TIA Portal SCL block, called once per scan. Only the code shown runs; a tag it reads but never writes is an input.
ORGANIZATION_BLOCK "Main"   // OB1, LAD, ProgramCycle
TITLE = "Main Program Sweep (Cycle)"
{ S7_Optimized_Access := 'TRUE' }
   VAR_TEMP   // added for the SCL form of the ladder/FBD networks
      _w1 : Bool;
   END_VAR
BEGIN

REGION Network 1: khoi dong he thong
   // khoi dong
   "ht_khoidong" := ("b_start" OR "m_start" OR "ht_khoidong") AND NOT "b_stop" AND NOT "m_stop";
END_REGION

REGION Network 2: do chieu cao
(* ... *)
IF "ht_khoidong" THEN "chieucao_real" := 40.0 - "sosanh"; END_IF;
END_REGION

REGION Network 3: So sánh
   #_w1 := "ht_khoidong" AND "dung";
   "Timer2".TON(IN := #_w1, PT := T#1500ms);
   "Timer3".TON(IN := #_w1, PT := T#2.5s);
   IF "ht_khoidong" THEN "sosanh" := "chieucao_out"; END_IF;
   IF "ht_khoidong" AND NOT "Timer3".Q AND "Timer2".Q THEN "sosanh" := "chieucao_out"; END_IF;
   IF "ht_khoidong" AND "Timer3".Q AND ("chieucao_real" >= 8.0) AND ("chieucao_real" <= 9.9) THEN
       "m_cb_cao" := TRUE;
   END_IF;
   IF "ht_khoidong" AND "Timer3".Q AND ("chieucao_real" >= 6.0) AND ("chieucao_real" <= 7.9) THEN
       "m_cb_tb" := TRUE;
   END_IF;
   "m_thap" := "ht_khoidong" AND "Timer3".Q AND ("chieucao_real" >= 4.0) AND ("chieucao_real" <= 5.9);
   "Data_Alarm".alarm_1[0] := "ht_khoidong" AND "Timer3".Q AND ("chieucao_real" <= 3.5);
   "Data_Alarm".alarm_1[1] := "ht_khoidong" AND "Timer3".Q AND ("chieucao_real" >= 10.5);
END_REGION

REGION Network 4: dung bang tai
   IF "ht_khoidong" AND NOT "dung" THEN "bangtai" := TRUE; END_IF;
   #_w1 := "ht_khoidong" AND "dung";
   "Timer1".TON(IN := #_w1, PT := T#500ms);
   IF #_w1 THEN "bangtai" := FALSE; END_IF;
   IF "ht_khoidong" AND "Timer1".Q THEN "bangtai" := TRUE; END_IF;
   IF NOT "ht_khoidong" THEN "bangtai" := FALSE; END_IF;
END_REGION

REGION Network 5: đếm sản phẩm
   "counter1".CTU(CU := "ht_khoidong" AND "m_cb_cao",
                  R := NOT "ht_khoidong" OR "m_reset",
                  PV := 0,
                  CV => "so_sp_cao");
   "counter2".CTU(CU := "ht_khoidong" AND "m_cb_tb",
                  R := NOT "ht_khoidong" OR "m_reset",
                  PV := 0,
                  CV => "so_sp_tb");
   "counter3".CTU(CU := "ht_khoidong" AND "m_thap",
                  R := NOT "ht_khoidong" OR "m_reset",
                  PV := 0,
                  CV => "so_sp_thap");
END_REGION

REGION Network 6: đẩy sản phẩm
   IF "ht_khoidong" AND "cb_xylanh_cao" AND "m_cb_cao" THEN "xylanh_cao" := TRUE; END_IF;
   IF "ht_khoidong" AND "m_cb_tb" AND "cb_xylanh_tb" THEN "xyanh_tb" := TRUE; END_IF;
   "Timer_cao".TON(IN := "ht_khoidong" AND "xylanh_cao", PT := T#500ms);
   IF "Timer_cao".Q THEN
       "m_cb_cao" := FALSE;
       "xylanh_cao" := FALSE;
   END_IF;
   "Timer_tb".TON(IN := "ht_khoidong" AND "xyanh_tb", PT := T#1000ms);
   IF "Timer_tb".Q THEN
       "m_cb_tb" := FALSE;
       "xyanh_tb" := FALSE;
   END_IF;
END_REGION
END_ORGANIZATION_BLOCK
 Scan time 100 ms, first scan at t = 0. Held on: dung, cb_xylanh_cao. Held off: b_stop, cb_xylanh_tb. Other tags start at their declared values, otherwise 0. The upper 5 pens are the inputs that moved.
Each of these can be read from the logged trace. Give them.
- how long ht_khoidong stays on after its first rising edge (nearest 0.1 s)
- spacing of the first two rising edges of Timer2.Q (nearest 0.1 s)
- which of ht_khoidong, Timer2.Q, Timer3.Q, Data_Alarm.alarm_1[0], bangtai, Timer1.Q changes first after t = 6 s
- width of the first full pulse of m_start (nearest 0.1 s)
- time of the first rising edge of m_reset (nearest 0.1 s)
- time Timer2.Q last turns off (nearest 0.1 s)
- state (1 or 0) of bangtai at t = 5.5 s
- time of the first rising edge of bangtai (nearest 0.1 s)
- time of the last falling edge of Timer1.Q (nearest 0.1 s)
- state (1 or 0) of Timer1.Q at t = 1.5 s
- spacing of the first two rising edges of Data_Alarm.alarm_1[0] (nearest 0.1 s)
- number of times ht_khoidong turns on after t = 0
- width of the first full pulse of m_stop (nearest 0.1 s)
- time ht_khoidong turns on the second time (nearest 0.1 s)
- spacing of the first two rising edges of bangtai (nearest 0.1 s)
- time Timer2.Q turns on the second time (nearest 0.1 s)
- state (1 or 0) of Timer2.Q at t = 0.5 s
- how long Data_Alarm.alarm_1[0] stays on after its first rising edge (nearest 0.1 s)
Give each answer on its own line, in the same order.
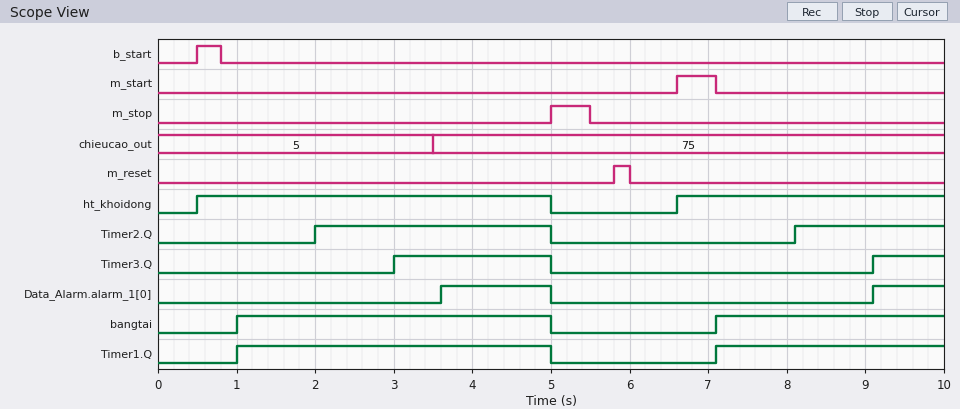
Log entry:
4.5 s
6.1 s
ht_khoidong
0.5 s
5.8 s
5.0 s
0
1.0 s
5.0 s
1
5.5 s
2
0.5 s
6.6 s
6.1 s
8.1 s
0
1.4 s
